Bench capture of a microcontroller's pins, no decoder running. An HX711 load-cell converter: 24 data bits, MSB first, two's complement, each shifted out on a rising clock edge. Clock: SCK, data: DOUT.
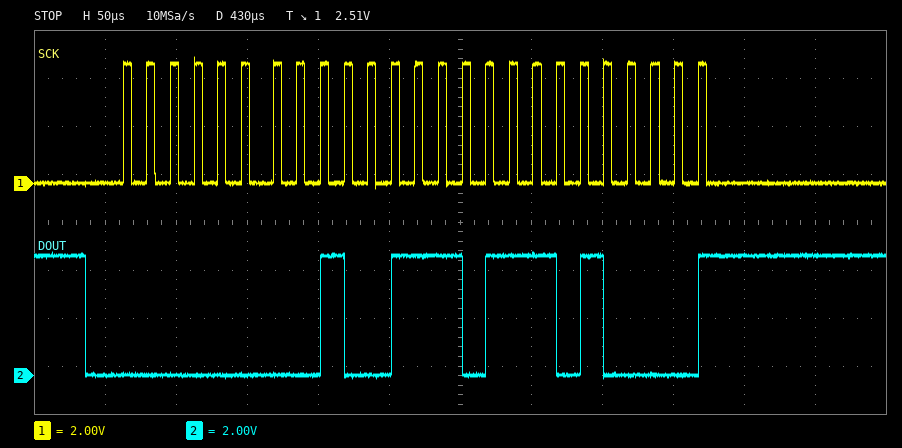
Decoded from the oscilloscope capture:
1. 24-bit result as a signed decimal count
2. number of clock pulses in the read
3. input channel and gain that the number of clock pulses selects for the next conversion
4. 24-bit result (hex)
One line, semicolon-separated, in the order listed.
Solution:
40400; 25; channel A, gain 128; 0x009DD0
